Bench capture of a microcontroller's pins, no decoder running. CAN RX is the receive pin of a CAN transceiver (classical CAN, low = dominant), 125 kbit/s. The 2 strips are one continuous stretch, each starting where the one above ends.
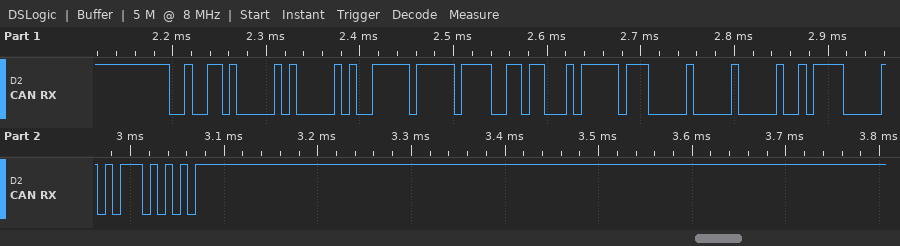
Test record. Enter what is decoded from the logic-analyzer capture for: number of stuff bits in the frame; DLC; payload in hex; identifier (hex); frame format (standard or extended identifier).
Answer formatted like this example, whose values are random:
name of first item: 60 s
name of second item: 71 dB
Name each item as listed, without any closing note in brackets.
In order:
number of stuff bits in the frame: 9
DLC: 8
payload in hex: 13 FF F3 62 FF 00 00 5E
identifier: 0x268
frame format: standard
